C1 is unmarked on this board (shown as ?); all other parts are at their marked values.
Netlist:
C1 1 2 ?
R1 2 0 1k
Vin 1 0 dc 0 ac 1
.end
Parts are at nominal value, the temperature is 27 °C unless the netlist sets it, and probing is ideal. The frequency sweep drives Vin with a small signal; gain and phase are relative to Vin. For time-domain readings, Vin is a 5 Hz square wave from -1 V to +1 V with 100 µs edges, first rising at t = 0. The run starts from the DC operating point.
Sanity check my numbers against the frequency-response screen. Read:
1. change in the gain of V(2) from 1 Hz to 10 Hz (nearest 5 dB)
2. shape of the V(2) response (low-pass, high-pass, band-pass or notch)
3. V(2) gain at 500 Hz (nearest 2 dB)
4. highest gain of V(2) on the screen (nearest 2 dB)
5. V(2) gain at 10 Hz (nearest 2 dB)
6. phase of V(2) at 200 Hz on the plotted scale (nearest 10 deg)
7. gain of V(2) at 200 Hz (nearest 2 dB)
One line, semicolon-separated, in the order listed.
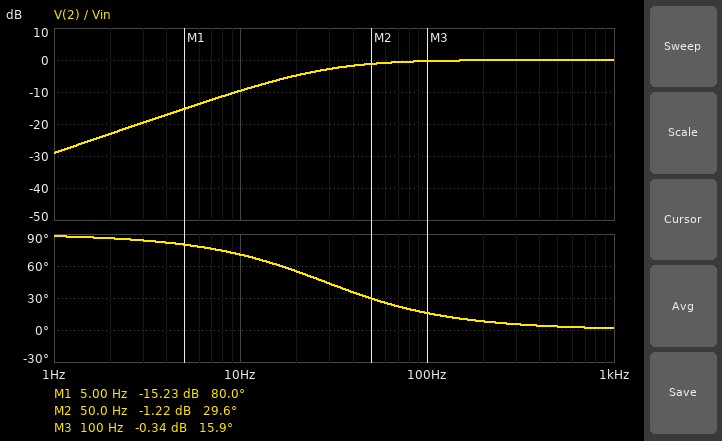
20 dB; high-pass; 0 dB; 0 dB; -10 dB; 10 deg; 0 dB
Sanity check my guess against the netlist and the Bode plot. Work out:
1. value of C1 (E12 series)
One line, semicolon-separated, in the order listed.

5.6 µF
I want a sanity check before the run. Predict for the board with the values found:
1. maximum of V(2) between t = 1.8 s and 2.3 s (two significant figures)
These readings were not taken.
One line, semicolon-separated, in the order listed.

2.0 V
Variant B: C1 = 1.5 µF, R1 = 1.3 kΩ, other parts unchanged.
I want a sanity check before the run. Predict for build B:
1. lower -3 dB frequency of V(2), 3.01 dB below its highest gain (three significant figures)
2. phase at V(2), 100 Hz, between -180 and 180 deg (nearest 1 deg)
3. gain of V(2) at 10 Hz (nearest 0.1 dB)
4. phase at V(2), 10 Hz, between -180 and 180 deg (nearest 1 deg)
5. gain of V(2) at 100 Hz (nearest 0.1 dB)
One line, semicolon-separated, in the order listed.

81.6 Hz; 39 deg; -18.3 dB; 83 deg; -2.2 dB
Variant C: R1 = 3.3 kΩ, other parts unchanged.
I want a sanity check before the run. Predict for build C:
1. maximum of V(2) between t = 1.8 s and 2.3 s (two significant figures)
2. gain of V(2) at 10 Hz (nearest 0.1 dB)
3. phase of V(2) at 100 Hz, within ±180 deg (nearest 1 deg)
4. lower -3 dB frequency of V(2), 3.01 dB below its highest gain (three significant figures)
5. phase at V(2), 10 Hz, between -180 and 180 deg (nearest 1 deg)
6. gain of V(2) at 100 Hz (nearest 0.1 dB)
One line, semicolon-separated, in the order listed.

2.0 V; -2.4 dB; 5 deg; 8.61 Hz; 41 deg; 0 dB
